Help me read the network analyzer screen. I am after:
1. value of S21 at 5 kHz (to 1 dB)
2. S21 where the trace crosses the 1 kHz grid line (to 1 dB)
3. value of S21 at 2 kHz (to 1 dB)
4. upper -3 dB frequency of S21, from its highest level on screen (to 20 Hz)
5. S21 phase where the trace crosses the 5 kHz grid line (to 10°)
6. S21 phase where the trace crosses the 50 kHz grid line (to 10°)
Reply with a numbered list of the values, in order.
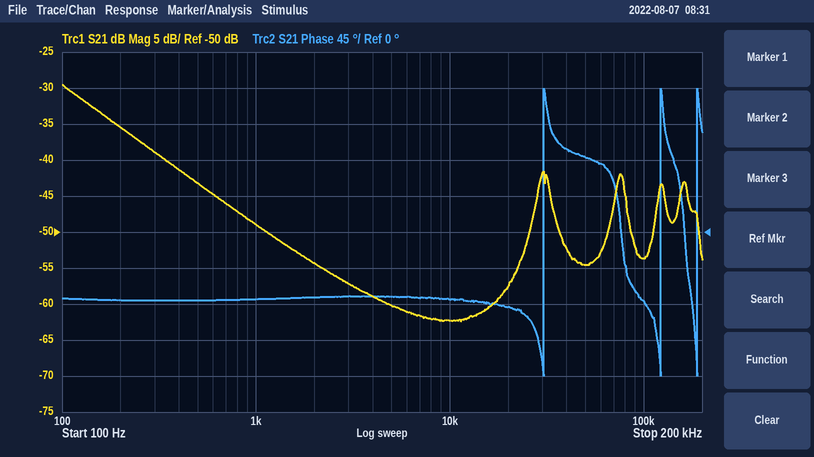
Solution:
1. -60 dB
2. -49 dB
3. -54 dB
4. 140 Hz
5. -80°
6. 90°
